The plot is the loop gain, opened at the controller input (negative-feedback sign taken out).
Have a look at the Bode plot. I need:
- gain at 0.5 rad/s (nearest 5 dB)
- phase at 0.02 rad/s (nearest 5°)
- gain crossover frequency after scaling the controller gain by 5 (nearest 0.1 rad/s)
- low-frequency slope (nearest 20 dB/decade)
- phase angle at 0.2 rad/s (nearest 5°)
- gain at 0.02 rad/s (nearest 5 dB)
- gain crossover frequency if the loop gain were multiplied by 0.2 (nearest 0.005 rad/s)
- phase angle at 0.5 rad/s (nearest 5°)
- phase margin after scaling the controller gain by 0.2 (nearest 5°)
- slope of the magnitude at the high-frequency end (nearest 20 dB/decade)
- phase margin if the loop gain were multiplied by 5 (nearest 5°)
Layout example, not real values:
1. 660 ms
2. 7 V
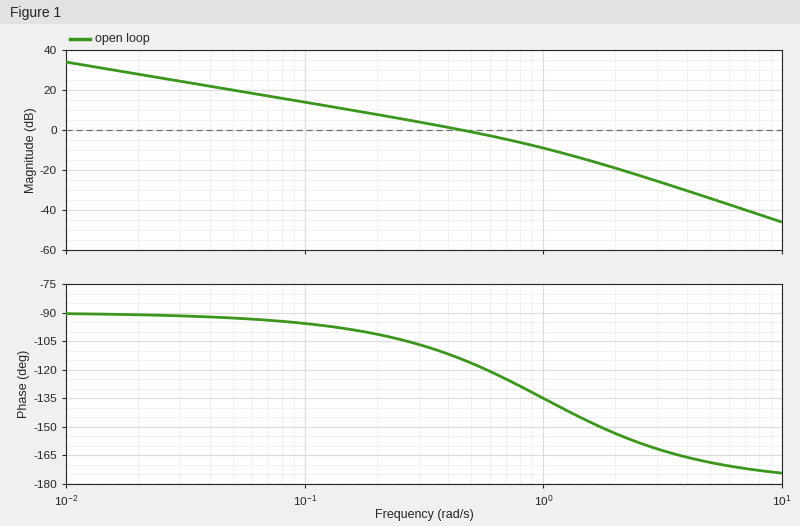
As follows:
1. 0 dB
2. -90°
3. 1.4 rad/s
4. -20 dB/decade
5. -100°
6. 30 dB
7. 0.100 rad/s
8. -115°
9. 85°
10. -40 dB/decade
11. 35°
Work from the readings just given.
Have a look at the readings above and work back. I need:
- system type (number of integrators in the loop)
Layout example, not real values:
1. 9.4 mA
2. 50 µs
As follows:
1. 1
